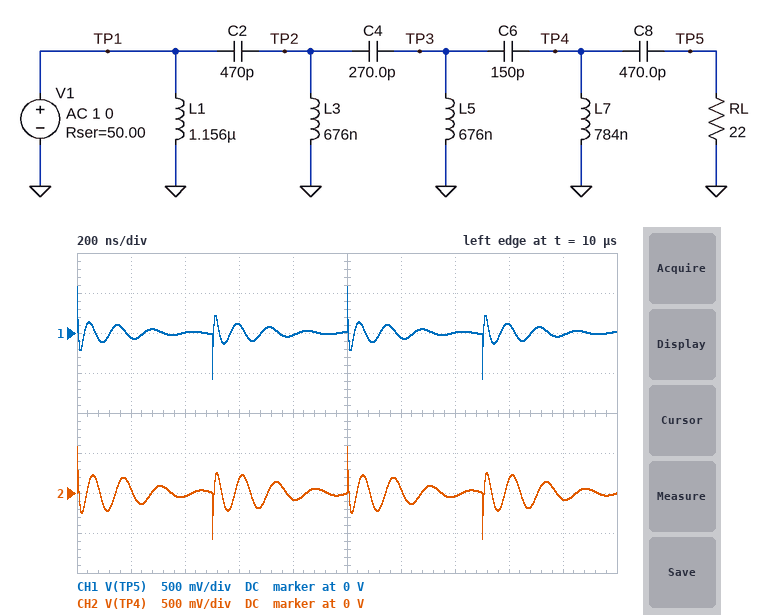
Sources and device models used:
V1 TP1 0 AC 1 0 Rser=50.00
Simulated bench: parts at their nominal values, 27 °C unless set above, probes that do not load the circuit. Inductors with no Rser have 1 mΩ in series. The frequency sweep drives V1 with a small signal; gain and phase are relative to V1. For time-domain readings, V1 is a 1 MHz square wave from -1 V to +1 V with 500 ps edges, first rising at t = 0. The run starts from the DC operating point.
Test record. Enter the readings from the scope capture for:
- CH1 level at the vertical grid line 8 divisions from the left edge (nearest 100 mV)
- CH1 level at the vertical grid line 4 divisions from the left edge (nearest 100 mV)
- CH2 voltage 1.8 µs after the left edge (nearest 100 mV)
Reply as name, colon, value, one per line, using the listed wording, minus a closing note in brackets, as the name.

CH1 level at the vertical grid line 8 divisions from the left edge: 100 mV
CH1 level at the vertical grid line 4 divisions from the left edge: 0 V
CH2 voltage 1.8 µs after the left edge: -100 mV
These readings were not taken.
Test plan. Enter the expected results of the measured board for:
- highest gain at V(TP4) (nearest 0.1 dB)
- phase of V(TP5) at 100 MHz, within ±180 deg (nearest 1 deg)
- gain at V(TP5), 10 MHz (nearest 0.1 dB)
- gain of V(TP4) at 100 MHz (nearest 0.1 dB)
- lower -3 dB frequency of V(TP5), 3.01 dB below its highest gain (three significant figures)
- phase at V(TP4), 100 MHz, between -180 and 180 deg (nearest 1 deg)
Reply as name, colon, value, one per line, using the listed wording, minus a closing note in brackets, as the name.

highest gain at V(TP4): -4.5 dB
phase of V(TP5) at 100 MHz, within ±180 deg: 26 deg
gain at V(TP5), 10 MHz: -10.5 dB
gain of V(TP4) at 100 MHz: -10.2 dB
lower -3 dB frequency of V(TP5), 3.01 dB below its highest gain: 7.05 MHz
phase at V(TP4), 100 MHz, between -180 and 180 deg: 17 deg
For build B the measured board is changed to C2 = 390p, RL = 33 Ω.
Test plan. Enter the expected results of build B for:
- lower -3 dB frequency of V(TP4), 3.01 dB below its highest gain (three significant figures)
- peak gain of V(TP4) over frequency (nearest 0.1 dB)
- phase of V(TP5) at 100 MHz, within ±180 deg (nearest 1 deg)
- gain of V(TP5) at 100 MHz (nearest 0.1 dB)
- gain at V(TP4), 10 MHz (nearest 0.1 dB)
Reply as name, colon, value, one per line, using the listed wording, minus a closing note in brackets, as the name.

lower -3 dB frequency of V(TP4), 3.01 dB below its highest gain: 6.78 MHz
peak gain of V(TP4) over frequency: -5.0 dB
phase of V(TP5) at 100 MHz, within ±180 deg: 26 deg
gain of V(TP5) at 100 MHz: -8.0 dB
gain at V(TP4), 10 MHz: -5.3 dB
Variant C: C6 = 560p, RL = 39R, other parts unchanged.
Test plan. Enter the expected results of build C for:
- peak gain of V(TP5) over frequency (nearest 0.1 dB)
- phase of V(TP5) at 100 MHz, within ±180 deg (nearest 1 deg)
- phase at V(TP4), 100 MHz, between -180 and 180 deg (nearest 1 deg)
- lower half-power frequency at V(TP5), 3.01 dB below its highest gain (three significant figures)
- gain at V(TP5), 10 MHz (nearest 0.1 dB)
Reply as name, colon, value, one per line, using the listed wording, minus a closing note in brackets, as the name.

peak gain of V(TP5) over frequency: -7.1 dB
phase of V(TP5) at 100 MHz, within ±180 deg: 20 deg
phase at V(TP4), 100 MHz, between -180 and 180 deg: 15 deg
lower half-power frequency at V(TP5), 3.01 dB below its highest gain: 7.97 MHz
gain at V(TP5), 10 MHz: -7.7 dB
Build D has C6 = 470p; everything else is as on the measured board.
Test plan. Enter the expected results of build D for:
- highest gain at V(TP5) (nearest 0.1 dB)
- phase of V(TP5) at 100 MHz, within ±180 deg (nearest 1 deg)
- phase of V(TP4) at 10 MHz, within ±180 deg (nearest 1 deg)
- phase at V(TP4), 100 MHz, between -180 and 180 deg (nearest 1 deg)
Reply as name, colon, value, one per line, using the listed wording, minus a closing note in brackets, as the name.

highest gain at V(TP5): -9.6 dB
phase of V(TP5) at 100 MHz, within ±180 deg: 20 deg
phase of V(TP4) at 10 MHz, within ±180 deg: 167 deg
phase at V(TP4), 100 MHz, between -180 and 180 deg: 11 deg
